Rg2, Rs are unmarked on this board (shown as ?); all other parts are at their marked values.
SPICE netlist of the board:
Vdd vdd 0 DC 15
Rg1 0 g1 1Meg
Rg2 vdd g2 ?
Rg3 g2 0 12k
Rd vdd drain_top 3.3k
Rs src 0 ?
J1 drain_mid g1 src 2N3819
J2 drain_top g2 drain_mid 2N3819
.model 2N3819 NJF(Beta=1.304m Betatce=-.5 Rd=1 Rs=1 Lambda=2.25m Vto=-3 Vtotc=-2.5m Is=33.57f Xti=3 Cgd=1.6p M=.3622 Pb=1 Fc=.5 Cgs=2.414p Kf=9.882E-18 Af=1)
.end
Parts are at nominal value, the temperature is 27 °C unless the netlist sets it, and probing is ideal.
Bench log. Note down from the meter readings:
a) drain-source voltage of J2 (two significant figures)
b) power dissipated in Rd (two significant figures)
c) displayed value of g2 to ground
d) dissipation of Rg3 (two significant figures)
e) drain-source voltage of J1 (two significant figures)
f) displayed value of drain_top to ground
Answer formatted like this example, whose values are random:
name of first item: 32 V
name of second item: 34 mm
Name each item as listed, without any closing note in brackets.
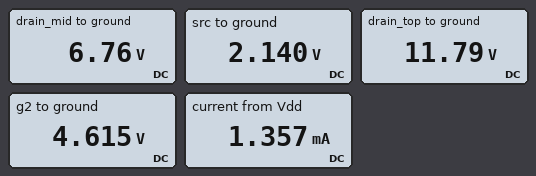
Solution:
drain-source voltage of J2: 5.0 V
power dissipated in Rd: 3.1 mW
displayed value of g2 to ground: 4.615 V
dissipation of Rg3: 1.8 mW
drain-source voltage of J1: 4.6 V
displayed value of drain_top to ground: 11.79 V
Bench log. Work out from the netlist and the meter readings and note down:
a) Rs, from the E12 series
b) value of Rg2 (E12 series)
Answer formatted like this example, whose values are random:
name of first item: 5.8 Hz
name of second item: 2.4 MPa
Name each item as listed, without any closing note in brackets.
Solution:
Rs, from the E12 series: 2.2 kΩ
value of Rg2: 27 kΩ
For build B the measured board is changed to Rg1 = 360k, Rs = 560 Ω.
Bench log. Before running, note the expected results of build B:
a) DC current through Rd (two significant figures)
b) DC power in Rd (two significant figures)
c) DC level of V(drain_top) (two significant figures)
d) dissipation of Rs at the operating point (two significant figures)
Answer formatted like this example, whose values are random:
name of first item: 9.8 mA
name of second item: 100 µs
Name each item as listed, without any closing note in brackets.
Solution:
DC current through Rd: 2.8 mA
DC power in Rd: 25 mW
DC level of V(drain_top): 5.9 V
dissipation of Rs at the operating point: 4.3 mW
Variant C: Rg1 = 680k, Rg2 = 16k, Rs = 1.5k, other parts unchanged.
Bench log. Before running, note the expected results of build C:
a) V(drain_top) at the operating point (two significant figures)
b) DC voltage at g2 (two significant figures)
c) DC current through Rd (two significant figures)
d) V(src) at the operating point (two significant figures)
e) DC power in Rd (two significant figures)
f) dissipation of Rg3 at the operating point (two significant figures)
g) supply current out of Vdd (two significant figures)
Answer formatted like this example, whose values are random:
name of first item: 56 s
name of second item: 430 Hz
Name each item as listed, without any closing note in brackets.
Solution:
V(drain_top) at the operating point: 11 V
DC voltage at g2: 6.4 V
DC current through Rd: 1.3 mA
V(src) at the operating point: 2.0 V
DC power in Rd: 5.8 mW
dissipation of Rg3 at the operating point: 3.4 mW
supply current out of Vdd: 1.9 mA
